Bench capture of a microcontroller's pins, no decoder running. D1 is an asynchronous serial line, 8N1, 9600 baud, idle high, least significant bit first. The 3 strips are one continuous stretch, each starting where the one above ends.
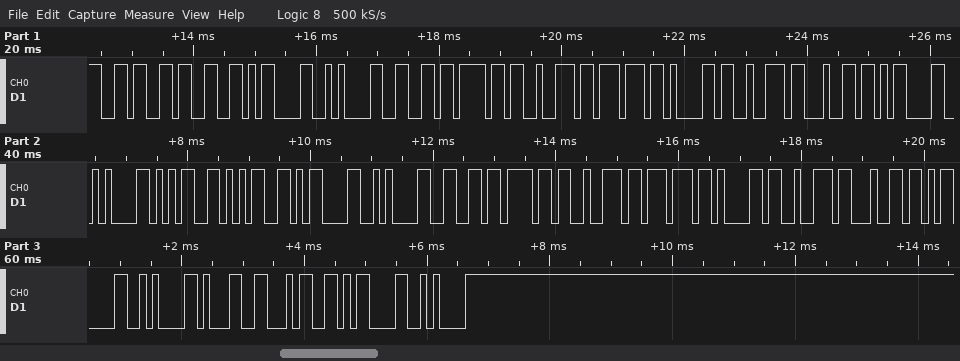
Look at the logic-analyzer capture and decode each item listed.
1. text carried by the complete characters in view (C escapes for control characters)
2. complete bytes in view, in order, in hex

"63\r\nforward\r\n55\r\nforward\r\n14\r\n"
0x36 0x33 0x0D 0x0A 0x66 0x6F 0x72 0x77 0x61 0x72 0x64 0x0D 0x0A 0x35 0x35 0x0D 0x0A 0x66 0x6F 0x72 0x77 0x61 0x72 0x64 0x0D 0x0A 0x31 0x34 0x0D 0x0A
